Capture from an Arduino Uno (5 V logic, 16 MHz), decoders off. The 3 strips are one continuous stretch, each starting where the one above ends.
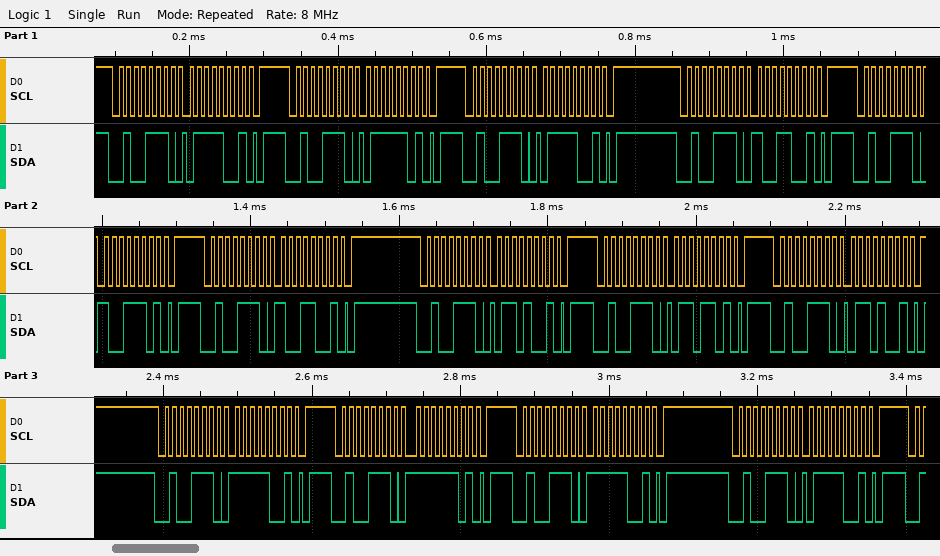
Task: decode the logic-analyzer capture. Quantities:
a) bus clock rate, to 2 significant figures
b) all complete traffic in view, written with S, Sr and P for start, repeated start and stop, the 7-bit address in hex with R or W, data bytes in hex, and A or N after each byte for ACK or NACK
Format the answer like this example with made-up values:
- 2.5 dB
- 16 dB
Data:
- 100 kHz
- S 27W A 79 A P S 27W A 7D A P S 27W A 79 A P S 27W A 99 A P S 27W A 9D A P S 27W A 99 A P S 27W A 69 A P S 27W A 6D A P S 27W A 69 A P S 27W A F9 A P S 27W A FD A P S 27W A F9 A P S 27W A 79 A P
